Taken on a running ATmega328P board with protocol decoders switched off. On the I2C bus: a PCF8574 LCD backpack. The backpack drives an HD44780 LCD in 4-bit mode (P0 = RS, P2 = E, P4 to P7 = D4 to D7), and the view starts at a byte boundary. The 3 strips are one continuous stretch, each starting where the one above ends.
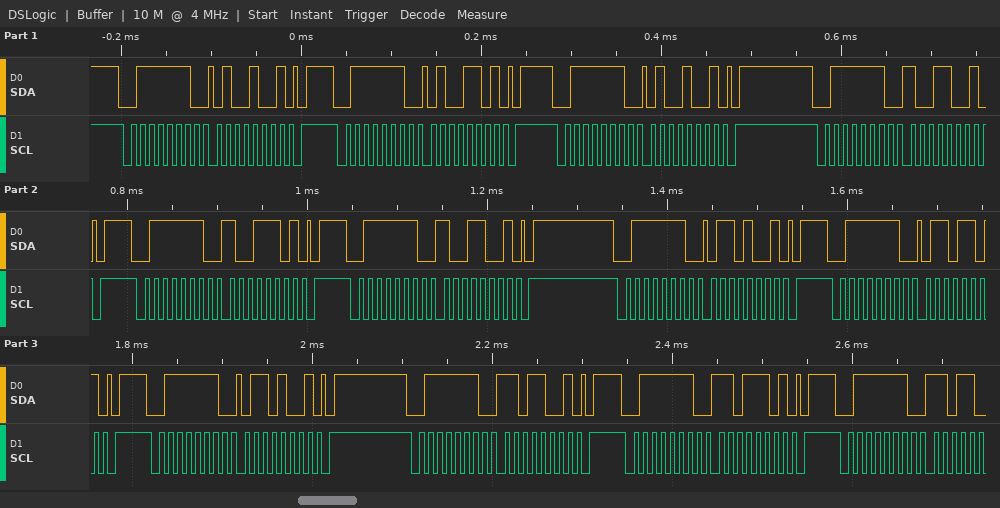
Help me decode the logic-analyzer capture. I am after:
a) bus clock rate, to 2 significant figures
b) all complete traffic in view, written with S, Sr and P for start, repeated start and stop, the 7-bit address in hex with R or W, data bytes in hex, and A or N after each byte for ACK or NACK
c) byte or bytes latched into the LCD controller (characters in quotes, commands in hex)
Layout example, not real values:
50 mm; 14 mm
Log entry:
100 kHz; S 3FW A 49 A P S 3FW A 4D A P S 3FW A 49 A P S 3FW A 99 A P S 3FW A 9D A P S 3FW A 99 A P S 3FW A 69 A P S 3FW A 6D A P S 3FW A 69 A P S 3FW A D9 A P S 3FW A DD A P S 3FW A; 'I'
